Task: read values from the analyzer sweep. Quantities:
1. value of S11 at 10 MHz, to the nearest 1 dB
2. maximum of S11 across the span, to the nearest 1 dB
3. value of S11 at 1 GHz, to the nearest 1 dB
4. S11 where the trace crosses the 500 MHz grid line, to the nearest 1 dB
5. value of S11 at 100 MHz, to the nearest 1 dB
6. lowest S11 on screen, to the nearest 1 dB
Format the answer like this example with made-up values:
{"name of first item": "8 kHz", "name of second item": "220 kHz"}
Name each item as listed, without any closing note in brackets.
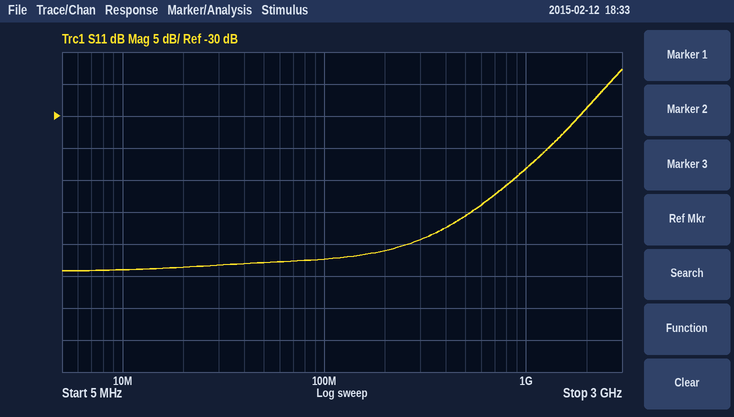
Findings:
{"value of S11 at 10 MHz, to the nearest 1 dB": "-54 dB", "maximum of S11 across the span, to the nearest 1 dB": "-23 dB", "value of S11 at 1 GHz, to the nearest 1 dB": "-38 dB", "S11 where the trace crosses the 500 MHz grid line, to the nearest 1 dB": "-46 dB", "value of S11 at 100 MHz, to the nearest 1 dB": "-52 dB", "lowest S11 on screen, to the nearest 1 dB": "-54 dB"}
